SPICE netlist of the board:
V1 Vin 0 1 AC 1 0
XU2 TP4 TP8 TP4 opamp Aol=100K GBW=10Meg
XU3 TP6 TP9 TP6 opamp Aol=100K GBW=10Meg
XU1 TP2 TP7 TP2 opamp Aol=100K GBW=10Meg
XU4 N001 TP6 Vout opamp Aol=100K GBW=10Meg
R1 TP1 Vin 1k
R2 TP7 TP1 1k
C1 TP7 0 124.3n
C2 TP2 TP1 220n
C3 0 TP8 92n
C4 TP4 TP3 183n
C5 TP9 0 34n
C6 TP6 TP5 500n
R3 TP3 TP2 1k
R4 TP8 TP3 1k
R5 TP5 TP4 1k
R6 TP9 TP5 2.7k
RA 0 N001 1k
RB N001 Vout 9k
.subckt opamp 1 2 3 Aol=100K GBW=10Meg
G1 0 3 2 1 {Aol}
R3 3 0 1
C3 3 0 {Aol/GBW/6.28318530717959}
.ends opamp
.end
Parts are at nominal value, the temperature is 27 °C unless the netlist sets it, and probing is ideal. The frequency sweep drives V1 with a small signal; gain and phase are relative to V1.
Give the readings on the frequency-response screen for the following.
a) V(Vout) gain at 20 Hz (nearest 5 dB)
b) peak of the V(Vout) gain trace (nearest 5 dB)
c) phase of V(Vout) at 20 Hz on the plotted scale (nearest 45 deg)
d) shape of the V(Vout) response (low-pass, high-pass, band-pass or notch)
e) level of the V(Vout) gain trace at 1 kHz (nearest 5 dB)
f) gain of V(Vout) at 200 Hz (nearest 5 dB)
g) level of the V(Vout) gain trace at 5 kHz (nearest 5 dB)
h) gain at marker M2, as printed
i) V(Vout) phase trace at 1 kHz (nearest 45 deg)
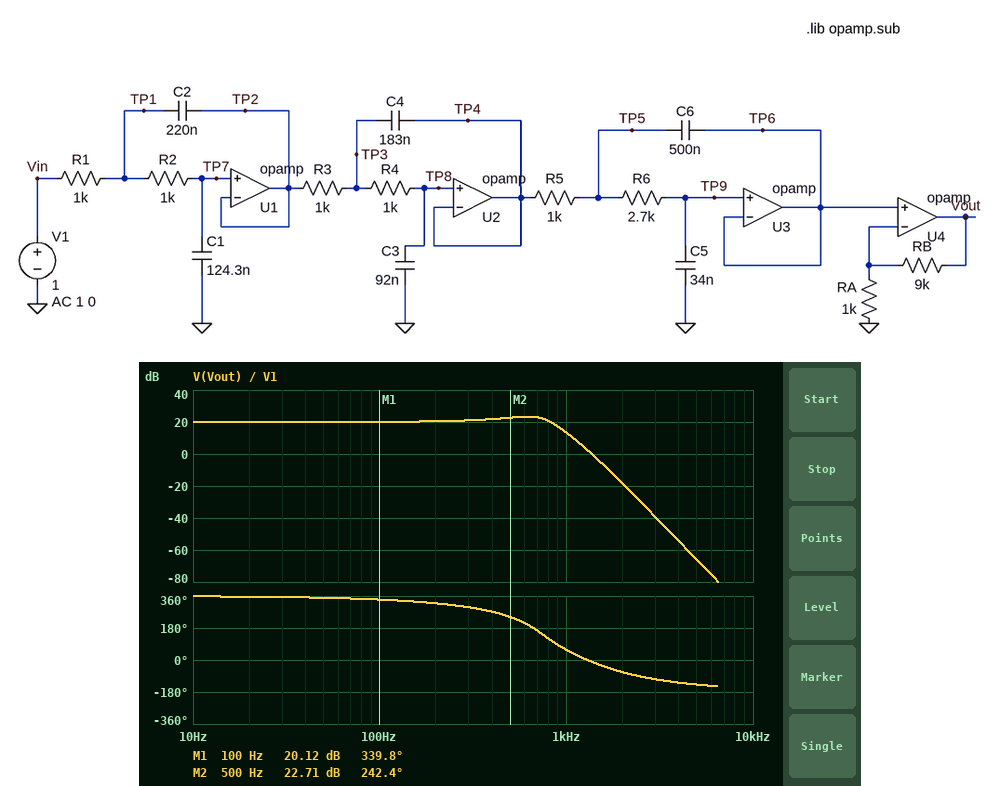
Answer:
20 dB
25 dB
360 deg
low-pass
15 dB
20 dB
-65 dB
22.71 dB
45 deg
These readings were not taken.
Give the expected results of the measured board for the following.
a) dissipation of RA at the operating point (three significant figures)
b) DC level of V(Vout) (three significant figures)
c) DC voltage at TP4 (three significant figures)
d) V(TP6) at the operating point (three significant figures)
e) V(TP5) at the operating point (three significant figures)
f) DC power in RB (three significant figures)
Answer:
1.00 mW
10.0 V
1.00 V
1.00 V
1.00 V
9.00 mW
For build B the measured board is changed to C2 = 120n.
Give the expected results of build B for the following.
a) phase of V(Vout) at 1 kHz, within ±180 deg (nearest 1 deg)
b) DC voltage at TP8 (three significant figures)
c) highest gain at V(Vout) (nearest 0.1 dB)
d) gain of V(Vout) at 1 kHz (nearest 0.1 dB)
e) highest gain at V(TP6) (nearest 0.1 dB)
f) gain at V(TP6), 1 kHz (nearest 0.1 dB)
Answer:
75 deg
1.00 V
22.6 dB
13.1 dB
2.6 dB
-6.9 dB
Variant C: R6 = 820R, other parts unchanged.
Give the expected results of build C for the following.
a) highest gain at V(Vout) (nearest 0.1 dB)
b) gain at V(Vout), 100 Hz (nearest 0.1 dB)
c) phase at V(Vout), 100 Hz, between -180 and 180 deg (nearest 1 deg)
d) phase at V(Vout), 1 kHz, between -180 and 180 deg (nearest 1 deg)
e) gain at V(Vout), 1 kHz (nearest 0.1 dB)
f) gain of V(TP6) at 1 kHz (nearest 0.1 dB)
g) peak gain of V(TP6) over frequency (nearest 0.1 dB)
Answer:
20.4 dB
20.0 dB
-18 deg
152 deg
19.0 dB
-1.0 dB
0.4 dB
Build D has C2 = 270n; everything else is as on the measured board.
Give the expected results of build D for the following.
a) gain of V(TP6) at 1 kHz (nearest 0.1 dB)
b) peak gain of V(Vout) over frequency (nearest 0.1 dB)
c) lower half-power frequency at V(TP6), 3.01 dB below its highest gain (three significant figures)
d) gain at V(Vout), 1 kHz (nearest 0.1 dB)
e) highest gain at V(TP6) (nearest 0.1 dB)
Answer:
-6.8 dB
23.8 dB
239 Hz
13.2 dB
3.8 dB
